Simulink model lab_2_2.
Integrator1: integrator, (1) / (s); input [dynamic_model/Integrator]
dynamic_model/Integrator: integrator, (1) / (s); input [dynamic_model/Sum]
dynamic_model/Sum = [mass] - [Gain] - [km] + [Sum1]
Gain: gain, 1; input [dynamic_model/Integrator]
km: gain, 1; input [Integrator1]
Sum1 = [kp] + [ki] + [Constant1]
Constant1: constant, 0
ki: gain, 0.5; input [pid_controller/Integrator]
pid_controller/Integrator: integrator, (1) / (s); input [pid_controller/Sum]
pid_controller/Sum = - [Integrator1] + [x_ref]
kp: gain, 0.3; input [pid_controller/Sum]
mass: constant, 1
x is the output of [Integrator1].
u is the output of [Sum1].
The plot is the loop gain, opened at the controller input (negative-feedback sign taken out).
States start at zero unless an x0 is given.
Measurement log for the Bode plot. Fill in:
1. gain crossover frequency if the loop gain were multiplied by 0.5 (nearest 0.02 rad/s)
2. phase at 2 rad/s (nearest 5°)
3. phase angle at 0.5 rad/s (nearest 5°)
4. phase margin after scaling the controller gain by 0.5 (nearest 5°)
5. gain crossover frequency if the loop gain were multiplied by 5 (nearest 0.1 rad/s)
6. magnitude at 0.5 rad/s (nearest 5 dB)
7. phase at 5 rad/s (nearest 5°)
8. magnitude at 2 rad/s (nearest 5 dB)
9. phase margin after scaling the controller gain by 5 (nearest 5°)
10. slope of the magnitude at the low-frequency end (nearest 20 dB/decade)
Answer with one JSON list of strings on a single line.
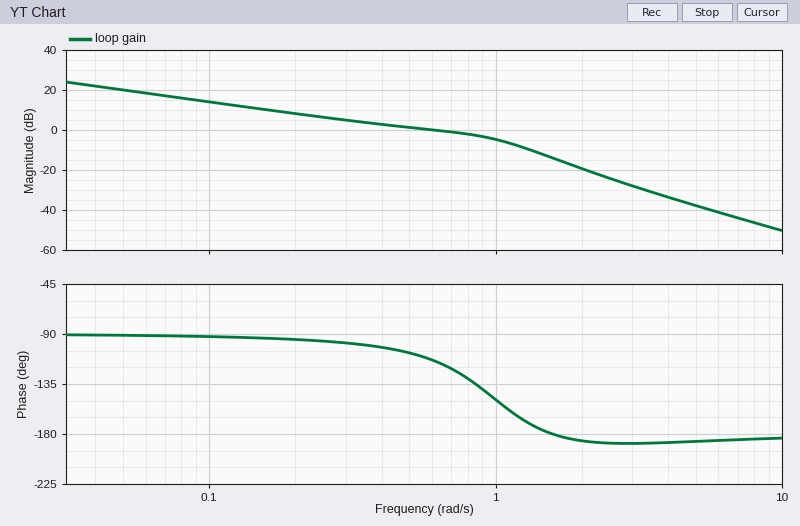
["0.26 rad/s", "-185°", "-105°", "85°", "1.6 rad/s", "0 dB", "-185°", "-20 dB", "0°", "-20 dB/decade"]
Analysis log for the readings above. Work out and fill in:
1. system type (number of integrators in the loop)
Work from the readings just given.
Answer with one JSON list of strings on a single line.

["1"]
